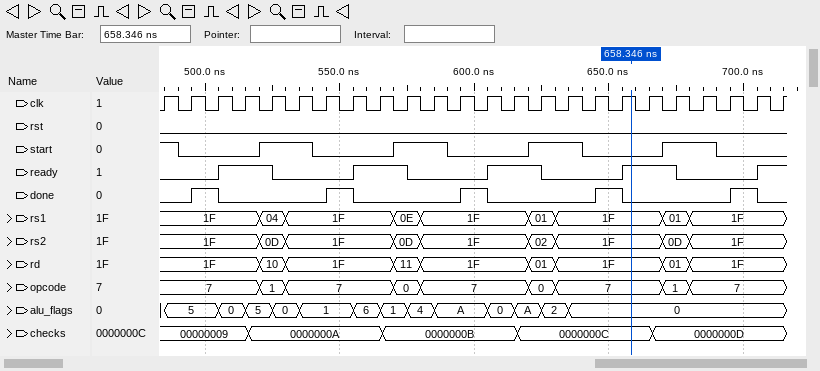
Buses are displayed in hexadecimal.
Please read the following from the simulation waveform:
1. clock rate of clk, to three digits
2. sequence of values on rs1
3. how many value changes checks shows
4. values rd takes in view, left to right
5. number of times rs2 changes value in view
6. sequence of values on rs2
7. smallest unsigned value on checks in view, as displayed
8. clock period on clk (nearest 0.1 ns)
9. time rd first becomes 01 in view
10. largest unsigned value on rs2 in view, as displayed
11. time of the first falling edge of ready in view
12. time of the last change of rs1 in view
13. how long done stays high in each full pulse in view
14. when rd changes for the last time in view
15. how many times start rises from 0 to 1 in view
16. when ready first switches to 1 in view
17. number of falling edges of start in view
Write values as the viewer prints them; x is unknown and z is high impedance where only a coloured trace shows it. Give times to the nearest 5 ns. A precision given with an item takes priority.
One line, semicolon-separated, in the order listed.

100 MHz; 1F, 04, 1F, 0E, 1F, 01, 1F, 01, 1F; 4; 1F, 10, 1F, 11, 1F, 01, 1F, 01, 1F; 8; 1F, 0D, 1F, 0D, 1F, 02, 1F, 0D, 1F; 00000009; 10 ns; 620 ns; 1F; 525 ns; 680 ns; 10 ns, 10 ns, 10 ns, 10 ns, 10 ns; 680 ns; 4; 505 ns; 5
